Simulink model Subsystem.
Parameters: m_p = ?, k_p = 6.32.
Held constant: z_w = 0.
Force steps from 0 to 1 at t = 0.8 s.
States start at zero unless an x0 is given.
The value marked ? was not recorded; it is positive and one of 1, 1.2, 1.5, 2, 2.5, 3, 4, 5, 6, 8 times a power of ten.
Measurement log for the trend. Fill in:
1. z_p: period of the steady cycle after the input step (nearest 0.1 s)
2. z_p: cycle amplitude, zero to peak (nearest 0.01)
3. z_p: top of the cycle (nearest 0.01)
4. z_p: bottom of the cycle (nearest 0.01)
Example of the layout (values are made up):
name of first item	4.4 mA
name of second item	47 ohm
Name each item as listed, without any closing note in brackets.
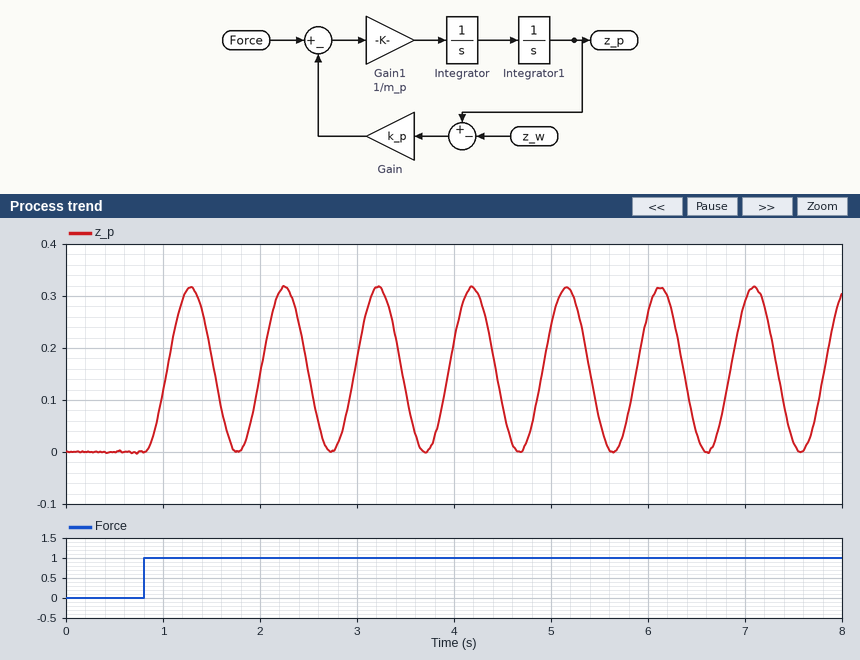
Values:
z_p: period of the steady cycle after the input step	1.0 s
z_p: cycle amplitude, zero to peak	0.16
z_p: top of the cycle	0.32
z_p: bottom of the cycle	0.00
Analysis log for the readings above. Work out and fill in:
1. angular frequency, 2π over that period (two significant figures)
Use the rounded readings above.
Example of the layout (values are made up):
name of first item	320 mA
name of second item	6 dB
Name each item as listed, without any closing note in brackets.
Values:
angular frequency, 2π over that period	6.3 rad/s
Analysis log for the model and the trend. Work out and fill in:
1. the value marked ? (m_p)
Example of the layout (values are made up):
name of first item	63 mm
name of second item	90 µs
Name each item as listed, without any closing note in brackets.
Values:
the value marked ?	0.15
